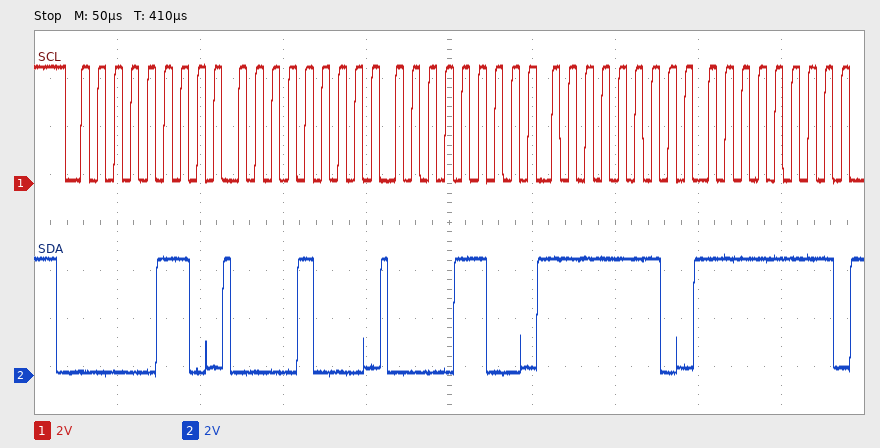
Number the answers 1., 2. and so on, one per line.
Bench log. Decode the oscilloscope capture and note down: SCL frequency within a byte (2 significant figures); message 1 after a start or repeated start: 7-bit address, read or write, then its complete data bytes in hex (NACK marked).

1. 100 kHz
2. 0x03 write: 08 0C FE FF
